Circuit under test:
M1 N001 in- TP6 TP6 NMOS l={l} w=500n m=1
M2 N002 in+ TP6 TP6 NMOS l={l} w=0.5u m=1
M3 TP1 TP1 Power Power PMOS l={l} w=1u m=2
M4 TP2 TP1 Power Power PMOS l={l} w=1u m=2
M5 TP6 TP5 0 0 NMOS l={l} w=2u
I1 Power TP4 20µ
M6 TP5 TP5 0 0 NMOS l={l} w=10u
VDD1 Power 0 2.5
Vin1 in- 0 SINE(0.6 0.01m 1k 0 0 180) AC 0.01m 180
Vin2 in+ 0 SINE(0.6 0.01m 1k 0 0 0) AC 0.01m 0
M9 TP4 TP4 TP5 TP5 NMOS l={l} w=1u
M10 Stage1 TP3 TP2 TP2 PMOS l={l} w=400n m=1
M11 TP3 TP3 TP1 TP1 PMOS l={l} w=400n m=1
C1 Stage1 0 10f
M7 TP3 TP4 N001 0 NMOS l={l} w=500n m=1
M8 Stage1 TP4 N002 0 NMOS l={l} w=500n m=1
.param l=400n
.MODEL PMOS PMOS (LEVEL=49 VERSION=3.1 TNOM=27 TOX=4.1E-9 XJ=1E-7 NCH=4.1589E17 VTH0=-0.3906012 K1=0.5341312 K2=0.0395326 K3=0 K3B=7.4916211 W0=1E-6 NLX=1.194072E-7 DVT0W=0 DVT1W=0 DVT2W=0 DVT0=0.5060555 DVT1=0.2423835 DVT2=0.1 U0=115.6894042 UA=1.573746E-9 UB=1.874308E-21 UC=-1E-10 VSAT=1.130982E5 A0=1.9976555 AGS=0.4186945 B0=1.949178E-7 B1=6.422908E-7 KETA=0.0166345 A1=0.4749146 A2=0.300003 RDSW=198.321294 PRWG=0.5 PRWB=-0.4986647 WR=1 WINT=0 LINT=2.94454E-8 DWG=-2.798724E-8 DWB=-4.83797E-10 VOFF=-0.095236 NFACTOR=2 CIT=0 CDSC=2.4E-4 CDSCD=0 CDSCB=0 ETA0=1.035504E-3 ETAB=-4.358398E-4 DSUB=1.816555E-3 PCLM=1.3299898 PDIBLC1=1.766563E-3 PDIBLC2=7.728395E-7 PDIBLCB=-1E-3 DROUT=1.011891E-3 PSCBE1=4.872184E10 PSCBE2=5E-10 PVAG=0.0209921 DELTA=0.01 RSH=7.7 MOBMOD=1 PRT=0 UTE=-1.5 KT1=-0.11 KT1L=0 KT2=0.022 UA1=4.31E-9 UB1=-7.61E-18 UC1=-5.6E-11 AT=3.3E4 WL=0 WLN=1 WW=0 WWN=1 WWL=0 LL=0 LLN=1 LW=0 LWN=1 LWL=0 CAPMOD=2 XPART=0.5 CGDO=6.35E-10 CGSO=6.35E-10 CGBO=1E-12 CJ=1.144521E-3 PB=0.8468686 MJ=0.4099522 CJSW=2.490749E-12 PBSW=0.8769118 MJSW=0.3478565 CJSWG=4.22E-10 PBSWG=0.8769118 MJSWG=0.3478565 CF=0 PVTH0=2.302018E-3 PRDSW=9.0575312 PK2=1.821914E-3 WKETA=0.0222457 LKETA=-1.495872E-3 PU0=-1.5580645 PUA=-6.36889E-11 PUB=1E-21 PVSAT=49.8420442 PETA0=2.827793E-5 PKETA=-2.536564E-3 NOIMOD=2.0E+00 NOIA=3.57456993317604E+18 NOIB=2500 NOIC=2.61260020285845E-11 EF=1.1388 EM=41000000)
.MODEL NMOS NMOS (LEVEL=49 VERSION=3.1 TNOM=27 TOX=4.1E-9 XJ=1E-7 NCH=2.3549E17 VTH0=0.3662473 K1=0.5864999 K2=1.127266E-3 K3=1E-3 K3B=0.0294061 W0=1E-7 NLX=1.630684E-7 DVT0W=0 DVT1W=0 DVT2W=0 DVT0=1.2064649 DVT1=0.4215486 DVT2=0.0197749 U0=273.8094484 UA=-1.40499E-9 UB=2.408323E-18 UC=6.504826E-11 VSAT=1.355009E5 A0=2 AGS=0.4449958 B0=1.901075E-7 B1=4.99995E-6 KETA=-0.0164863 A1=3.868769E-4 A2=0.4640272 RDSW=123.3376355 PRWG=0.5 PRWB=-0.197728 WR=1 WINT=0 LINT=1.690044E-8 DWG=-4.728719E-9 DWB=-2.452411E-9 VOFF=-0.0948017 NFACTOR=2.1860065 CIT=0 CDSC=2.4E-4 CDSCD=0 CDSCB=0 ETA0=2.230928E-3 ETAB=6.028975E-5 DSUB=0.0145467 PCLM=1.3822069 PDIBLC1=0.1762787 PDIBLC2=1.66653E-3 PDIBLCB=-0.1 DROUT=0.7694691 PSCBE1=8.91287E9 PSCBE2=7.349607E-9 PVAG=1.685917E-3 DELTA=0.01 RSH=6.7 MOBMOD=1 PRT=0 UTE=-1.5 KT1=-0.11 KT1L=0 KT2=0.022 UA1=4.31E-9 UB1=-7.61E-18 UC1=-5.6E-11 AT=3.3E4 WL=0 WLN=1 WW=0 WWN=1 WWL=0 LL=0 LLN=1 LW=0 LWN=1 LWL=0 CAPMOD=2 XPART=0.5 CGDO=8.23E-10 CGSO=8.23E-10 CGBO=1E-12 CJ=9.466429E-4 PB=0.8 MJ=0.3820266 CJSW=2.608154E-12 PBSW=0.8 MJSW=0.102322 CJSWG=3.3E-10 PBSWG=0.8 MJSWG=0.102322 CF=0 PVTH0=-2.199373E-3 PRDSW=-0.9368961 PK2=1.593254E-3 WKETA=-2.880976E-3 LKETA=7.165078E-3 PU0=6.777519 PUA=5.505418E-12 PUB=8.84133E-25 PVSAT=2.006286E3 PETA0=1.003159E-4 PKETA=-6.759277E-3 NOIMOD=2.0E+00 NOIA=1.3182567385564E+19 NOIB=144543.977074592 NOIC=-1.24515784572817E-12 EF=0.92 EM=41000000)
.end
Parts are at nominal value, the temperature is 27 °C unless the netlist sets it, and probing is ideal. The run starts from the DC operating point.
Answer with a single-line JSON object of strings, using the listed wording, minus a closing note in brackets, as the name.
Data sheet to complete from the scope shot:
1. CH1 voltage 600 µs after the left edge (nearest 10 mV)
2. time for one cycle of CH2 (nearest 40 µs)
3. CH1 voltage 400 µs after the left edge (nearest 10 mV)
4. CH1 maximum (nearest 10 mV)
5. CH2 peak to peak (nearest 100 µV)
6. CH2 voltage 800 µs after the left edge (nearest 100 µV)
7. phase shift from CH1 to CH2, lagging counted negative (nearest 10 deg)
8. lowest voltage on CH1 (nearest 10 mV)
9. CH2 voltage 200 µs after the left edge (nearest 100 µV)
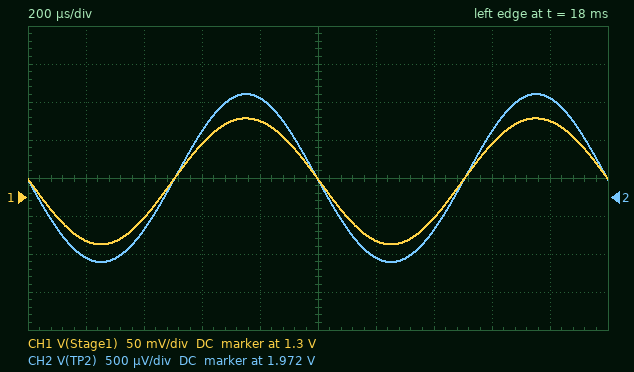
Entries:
{"CH1 voltage 600 µs after the left edge": "1.37 V", "time for one cycle of CH2": "1.00 ms", "CH1 voltage 400 µs after the left edge": "1.27 V", "CH1 maximum": "1.40 V", "CH2 peak to peak": "2.2 mV", "CH2 voltage 800 µs after the left edge": "1.9728 V", "phase shift from CH1 to CH2, lagging counted negative": "0 deg", "lowest voltage on CH1": "1.24 V", "CH2 voltage 200 µs after the left edge": "1.9707 V"}
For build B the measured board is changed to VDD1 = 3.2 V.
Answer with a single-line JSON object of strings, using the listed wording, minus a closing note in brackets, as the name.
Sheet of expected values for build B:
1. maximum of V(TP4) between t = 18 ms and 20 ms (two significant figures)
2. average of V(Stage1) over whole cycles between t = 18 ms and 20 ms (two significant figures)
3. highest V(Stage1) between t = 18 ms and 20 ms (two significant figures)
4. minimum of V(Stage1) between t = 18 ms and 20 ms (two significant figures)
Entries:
{"maximum of V(TP4) between t = 18 ms and 20 ms": "1.2 V", "average of V(Stage1) over whole cycles between t = 18 ms and 20 ms": "2.0 V", "highest V(Stage1) between t = 18 ms and 20 ms": "2.1 V", "minimum of V(Stage1) between t = 18 ms and 20 ms": "1.9 V"}
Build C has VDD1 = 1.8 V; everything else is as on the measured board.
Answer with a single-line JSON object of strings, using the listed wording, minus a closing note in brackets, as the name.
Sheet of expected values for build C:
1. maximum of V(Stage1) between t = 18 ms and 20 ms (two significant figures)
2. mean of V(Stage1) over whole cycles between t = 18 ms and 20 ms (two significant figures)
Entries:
{"maximum of V(Stage1) between t = 18 ms and 20 ms": "630 mV", "mean of V(Stage1) over whole cycles between t = 18 ms and 20 ms": "620 mV"}
